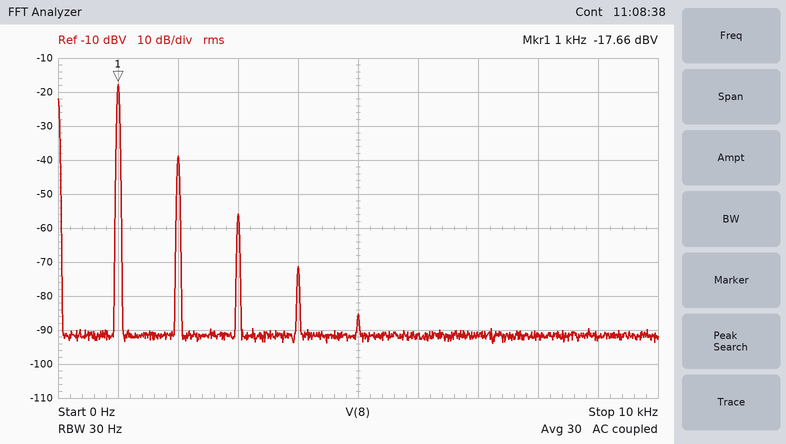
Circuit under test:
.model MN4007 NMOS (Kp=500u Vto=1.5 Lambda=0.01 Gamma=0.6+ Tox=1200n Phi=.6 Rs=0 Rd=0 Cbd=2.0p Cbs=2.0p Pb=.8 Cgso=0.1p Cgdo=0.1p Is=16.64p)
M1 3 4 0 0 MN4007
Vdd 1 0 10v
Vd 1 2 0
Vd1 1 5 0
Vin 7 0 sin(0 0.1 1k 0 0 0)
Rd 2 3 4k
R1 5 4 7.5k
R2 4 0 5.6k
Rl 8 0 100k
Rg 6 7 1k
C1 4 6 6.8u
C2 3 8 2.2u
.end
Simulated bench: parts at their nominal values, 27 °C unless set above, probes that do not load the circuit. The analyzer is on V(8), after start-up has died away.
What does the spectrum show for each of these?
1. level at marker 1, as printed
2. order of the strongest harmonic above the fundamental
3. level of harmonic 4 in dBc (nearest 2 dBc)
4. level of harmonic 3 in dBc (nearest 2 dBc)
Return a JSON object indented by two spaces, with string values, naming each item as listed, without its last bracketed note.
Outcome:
{
  "level at marker 1, as printed": "-17.66 dBV",
  "order of the strongest harmonic above the fundamental": "2",
  "level of harmonic 4 in dBc": "-54 dBc",
  "level of harmonic 3 in dBc": "-38 dBc"
}
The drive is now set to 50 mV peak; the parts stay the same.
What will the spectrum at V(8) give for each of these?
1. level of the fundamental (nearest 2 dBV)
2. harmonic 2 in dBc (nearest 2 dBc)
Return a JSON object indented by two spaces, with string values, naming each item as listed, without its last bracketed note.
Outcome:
{
  "level of the fundamental": "-24 dBV",
  "harmonic 2 in dBc": "-28 dBc"
}
